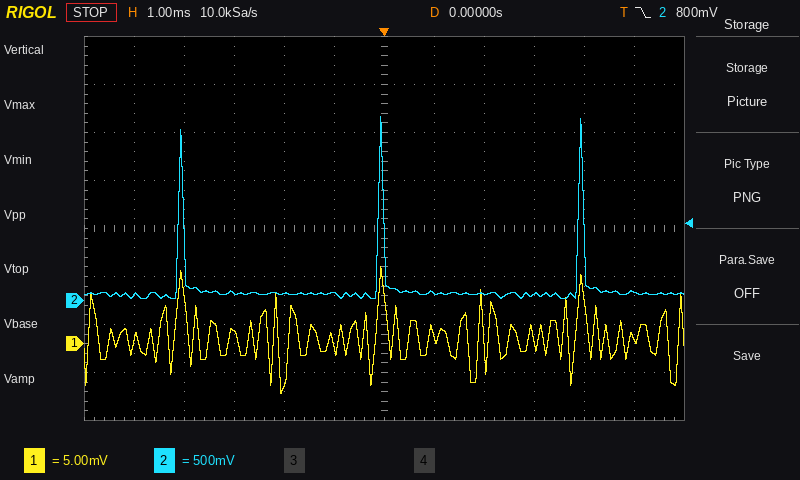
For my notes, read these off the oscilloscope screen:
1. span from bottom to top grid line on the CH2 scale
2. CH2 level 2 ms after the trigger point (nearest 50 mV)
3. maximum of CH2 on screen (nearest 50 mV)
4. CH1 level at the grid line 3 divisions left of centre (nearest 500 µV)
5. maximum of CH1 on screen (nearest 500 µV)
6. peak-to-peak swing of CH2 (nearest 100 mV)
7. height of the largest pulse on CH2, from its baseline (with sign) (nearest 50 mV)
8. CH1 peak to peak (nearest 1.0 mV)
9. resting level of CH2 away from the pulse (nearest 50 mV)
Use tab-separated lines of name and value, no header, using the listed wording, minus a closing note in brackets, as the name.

span from bottom to top grid line on the CH2 scale	4 V
CH2 level 2 ms after the trigger point	50 mV
maximum of CH2 on screen	1.90 V
CH1 level at the grid line 3 divisions left of centre	1.0 mV
maximum of CH1 on screen	8.0 mV
peak-to-peak swing of CH2	1.90 V
height of the largest pulse on CH2, from its baseline (with sign)	+1.85 V
CH1 peak to peak	13.0 mV
resting level of CH2 away from the pulse	50 mV
